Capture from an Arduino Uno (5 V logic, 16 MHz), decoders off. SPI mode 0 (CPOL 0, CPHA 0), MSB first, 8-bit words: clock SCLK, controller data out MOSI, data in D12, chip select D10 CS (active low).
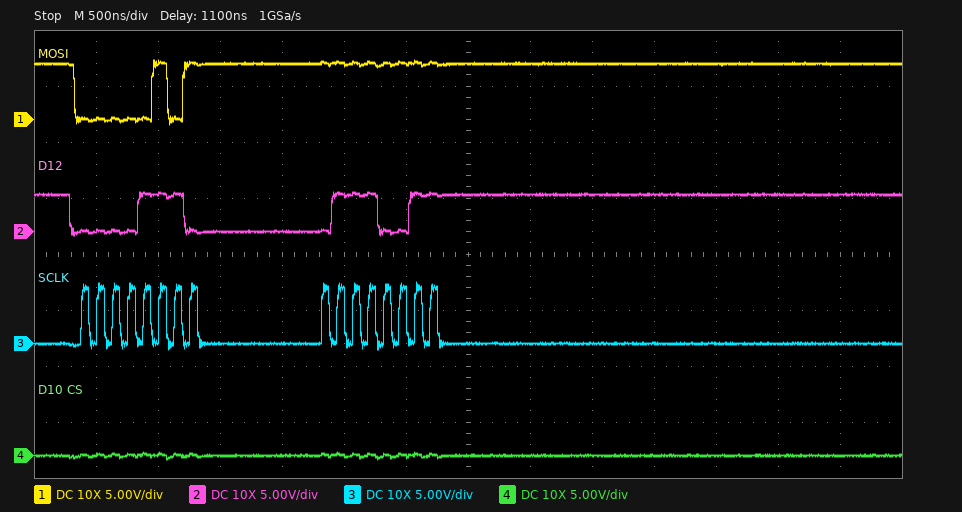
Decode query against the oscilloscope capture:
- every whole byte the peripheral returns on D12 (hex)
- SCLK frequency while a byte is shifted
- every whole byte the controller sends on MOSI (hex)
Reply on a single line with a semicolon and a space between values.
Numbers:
0E 73; 8 MHz; 05 FF
